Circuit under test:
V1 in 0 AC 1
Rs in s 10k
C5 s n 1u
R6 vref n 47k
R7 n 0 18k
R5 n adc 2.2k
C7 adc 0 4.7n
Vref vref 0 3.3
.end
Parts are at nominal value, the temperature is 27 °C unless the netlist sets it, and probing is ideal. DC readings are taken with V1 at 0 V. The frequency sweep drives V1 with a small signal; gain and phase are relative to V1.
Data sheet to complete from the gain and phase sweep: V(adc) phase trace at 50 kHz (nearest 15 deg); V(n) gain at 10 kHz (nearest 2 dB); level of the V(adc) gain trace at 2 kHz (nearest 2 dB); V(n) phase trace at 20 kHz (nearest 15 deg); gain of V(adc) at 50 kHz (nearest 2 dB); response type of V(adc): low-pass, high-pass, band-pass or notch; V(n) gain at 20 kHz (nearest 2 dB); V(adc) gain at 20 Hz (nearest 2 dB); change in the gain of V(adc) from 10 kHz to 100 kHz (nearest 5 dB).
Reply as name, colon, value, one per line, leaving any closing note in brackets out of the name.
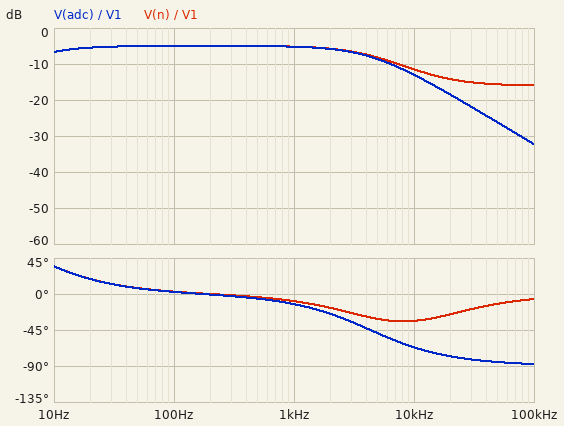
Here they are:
V(adc) phase trace at 50 kHz: -90 deg
V(n) gain at 10 kHz: -12 dB
level of the V(adc) gain trace at 2 kHz: -6 dB
V(n) phase trace at 20 kHz: -30 deg
gain of V(adc) at 50 kHz: -26 dB
response type of V(adc): low-pass, high-pass, band-pass or notch: low-pass
V(n) gain at 20 kHz: -14 dB
V(adc) gain at 20 Hz: -6 dB
change in the gain of V(adc) from 10 kHz to 100 kHz: -20 dB
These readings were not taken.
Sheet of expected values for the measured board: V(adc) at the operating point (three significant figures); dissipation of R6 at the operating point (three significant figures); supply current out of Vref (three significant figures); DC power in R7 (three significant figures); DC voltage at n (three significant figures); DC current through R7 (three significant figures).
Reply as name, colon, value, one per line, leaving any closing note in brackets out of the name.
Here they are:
V(adc) at the operating point: 914 mV
dissipation of R6 at the operating point: 121 µW
supply current out of Vref: 50.8 µA
DC power in R7: 46.4 µW
DC voltage at n: 914 mV
DC current through R7: 50.8 µA
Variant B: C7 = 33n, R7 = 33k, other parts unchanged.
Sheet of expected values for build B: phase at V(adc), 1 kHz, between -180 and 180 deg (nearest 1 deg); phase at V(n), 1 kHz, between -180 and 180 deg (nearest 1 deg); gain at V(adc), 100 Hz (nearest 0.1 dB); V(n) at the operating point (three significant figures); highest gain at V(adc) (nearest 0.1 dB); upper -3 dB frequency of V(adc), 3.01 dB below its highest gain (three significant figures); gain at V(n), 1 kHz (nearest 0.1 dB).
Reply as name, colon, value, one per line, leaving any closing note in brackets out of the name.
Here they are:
phase at V(adc), 1 kHz, between -180 and 180 deg: -61 deg
phase at V(n), 1 kHz, between -180 and 180 deg: -36 deg
gain at V(adc), 100 Hz: -3.9 dB
V(n) at the operating point: 1.36 V
highest gain at V(adc): -3.8 dB
upper -3 dB frequency of V(adc), 3.01 dB below its highest gain: 567 Hz
gain at V(n), 1 kHz: -9.2 dB
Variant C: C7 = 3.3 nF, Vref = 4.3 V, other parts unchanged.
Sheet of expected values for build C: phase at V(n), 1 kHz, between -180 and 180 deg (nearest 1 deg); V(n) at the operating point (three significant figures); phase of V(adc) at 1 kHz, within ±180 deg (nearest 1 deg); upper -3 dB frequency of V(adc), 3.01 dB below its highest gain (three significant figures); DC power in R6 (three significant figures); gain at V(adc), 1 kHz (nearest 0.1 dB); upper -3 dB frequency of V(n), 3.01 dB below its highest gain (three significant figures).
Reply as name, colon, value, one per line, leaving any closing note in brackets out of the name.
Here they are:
phase at V(n), 1 kHz, between -180 and 180 deg: -6 deg
V(n) at the operating point: 1.19 V
phase of V(adc) at 1 kHz, within ±180 deg: -9 deg
upper -3 dB frequency of V(adc), 3.01 dB below its highest gain: 6.16 kHz
DC power in R6: 206 µW
gain at V(adc), 1 kHz: -5.1 dB
upper -3 dB frequency of V(n), 3.01 dB below its highest gain: 6.71 kHz
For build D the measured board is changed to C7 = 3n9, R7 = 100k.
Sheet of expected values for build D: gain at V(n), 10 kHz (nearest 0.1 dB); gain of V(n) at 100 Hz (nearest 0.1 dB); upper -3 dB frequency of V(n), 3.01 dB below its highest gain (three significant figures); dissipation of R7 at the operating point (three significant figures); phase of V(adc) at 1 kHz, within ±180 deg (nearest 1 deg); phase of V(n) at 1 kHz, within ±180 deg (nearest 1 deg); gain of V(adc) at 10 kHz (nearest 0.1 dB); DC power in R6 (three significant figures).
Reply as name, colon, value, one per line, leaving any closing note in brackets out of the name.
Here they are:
gain at V(n), 10 kHz: -9.6 dB
gain of V(n) at 100 Hz: -2.4 dB
upper -3 dB frequency of V(n), 3.01 dB below its highest gain: 4.40 kHz
dissipation of R7 at the operating point: 50.4 µW
phase of V(adc) at 1 kHz, within ±180 deg: -13 deg
phase of V(n) at 1 kHz, within ±180 deg: -10 deg
gain of V(adc) at 10 kHz: -10.7 dB
DC power in R6: 23.7 µW
